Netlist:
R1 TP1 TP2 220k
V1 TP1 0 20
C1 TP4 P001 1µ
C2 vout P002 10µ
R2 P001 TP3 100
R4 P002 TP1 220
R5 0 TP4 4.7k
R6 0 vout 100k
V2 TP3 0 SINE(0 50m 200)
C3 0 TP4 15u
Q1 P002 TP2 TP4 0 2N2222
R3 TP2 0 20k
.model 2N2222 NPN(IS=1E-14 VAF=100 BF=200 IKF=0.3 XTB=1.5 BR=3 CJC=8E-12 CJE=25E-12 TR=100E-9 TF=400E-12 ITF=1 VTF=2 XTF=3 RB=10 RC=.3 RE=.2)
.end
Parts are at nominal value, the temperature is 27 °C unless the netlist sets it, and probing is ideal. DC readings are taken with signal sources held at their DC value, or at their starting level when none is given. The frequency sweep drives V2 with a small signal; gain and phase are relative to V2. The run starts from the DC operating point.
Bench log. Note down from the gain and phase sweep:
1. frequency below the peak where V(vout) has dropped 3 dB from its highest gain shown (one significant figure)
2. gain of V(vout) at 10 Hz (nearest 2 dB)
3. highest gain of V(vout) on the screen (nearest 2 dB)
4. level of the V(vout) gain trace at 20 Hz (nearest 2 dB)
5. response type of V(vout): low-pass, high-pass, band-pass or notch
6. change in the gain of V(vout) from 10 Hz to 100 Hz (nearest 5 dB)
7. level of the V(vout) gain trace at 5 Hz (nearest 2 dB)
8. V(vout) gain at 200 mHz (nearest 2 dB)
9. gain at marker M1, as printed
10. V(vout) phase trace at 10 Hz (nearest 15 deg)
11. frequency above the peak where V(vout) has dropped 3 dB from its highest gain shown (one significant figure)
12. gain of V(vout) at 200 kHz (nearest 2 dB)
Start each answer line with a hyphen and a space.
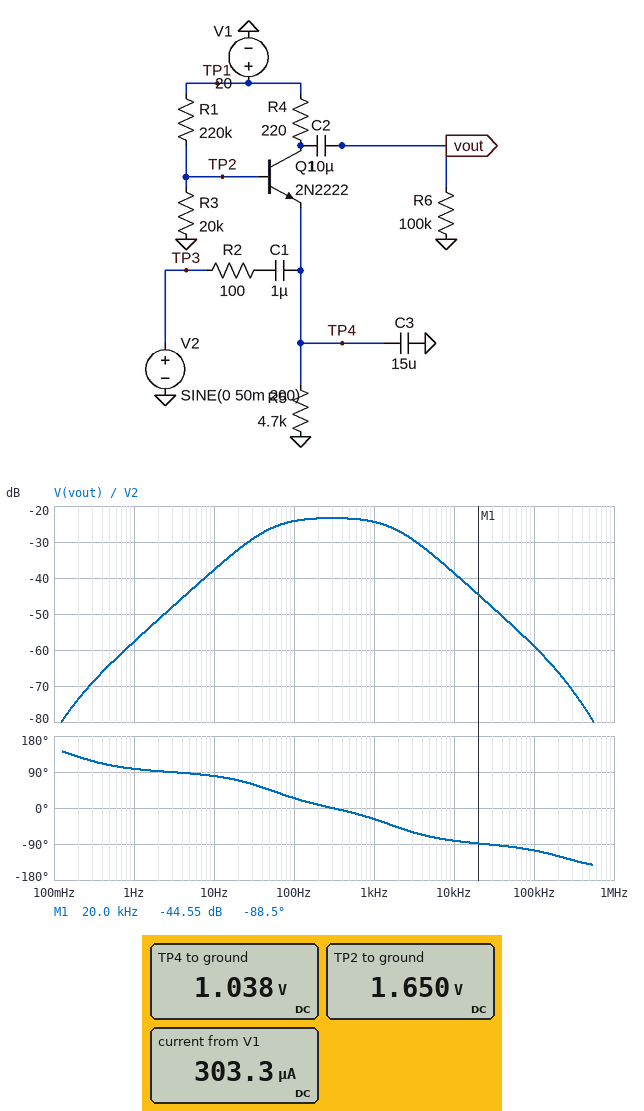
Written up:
- 50 Hz
- -38 dB
- -24 dB
- -32 dB
- band-pass
- 15 dB
- -44 dB
- -74 dB
- -44.55 dB
- 75 deg
- 2 kHz
- -66 dB
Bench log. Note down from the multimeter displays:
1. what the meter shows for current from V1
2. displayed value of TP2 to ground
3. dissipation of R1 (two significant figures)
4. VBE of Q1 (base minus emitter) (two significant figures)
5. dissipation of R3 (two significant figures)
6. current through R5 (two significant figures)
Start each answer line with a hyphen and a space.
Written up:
- 303.3 µA
- 1.650 V
- 1.5 mW
- 610 mV
- 140 µW
- 220 µA
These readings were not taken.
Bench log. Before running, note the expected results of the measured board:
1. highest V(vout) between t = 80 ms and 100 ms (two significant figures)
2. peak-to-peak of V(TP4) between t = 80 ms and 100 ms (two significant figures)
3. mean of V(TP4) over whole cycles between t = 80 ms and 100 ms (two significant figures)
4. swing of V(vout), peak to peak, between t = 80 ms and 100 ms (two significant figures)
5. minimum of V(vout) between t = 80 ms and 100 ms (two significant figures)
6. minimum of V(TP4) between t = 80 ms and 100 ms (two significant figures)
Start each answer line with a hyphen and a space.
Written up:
- 3.3 mV
- 6.0 mV
- 1.0 V
- 6.7 mV
- -3.4 mV
- 1.0 V
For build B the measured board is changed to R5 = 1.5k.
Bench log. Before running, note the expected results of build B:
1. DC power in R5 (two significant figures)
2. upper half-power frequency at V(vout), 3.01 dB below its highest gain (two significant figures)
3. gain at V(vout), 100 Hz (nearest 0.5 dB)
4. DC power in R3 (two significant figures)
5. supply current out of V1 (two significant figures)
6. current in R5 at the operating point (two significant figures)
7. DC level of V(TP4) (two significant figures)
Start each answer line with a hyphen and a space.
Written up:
- 640 µW
- 1.9 kHz
- -21.5 dB
- 130 µW
- 730 µA
- 650 µA
- 980 mV
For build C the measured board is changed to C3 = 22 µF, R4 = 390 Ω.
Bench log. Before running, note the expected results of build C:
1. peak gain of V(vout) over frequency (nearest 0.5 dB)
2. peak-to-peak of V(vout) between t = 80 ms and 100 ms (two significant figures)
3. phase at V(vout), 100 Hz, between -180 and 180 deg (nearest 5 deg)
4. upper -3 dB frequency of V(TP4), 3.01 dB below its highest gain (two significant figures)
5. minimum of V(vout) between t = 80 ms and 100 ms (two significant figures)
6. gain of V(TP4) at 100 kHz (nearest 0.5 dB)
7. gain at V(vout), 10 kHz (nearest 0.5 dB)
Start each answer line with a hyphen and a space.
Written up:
- -21.5 dB
- 8.4 mV
- 15 deg
- 1.7 kHz
- -4.2 mV
- -63.0 dB
- -37.0 dB
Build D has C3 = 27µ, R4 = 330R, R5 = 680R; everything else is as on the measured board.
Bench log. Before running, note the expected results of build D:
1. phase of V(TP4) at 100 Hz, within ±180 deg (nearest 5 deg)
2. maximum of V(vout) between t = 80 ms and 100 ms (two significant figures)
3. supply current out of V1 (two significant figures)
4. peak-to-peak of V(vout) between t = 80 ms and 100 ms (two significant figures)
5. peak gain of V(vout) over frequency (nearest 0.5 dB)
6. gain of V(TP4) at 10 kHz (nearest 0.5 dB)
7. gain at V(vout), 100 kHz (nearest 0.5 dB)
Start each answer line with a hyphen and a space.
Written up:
- 30 deg
- 5.6 mV
- 1.4 mA
- 11 mV
- -19.0 dB
- -44.5 dB
- -54.5 dB
